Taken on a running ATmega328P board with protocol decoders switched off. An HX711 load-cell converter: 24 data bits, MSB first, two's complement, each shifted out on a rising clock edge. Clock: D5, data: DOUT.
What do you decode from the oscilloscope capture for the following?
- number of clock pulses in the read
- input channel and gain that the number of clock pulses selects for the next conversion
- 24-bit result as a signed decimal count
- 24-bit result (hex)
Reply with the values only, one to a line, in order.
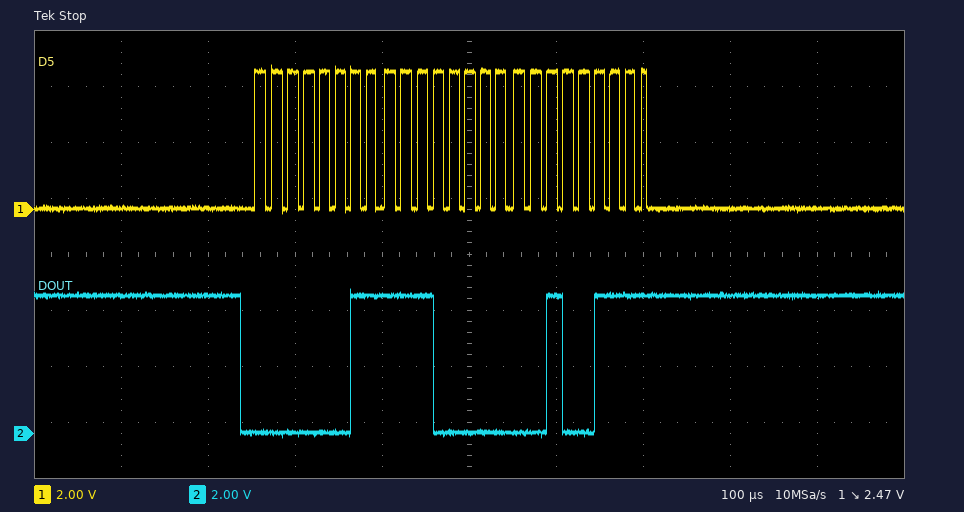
25
channel A, gain 128
253991
0x03E027
